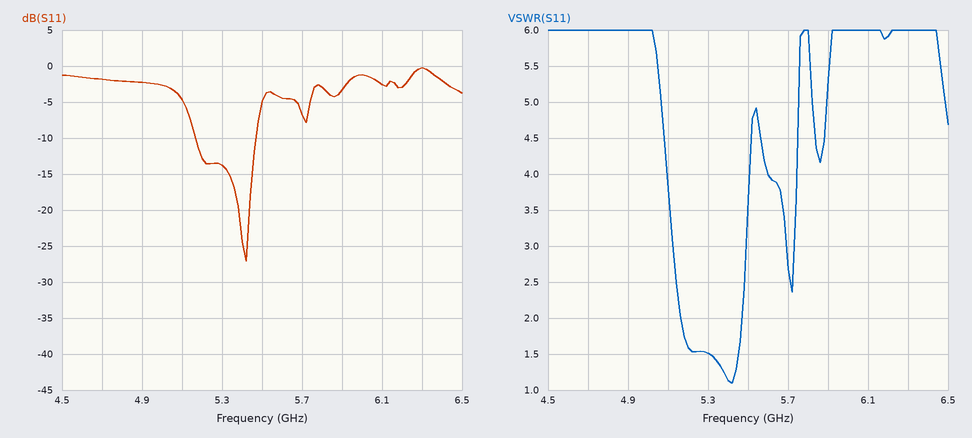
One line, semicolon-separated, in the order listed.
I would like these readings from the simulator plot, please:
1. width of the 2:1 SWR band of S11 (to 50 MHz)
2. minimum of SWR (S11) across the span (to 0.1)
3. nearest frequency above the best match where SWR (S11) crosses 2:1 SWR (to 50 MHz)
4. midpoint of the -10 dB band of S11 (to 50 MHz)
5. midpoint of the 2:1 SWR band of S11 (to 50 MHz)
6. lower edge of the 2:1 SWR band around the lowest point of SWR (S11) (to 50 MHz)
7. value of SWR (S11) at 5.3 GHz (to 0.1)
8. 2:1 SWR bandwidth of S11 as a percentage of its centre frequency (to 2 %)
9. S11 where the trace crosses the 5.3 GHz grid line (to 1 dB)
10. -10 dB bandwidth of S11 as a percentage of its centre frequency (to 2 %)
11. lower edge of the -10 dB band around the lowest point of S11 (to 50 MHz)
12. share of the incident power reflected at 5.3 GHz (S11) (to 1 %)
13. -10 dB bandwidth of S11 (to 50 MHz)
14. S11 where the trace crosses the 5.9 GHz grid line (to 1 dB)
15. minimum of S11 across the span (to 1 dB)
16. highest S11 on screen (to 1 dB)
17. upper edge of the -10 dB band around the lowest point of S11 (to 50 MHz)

300 MHz; 1.1; 5.45 GHz; 5.30 GHz; 5.30 GHz; 5.15 GHz; 1.5; 6 %; -14 dB; 6 %; 5.15 GHz; 4 %; 300 MHz; -3 dB; -27 dB; 0 dB; 5.45 GHz
